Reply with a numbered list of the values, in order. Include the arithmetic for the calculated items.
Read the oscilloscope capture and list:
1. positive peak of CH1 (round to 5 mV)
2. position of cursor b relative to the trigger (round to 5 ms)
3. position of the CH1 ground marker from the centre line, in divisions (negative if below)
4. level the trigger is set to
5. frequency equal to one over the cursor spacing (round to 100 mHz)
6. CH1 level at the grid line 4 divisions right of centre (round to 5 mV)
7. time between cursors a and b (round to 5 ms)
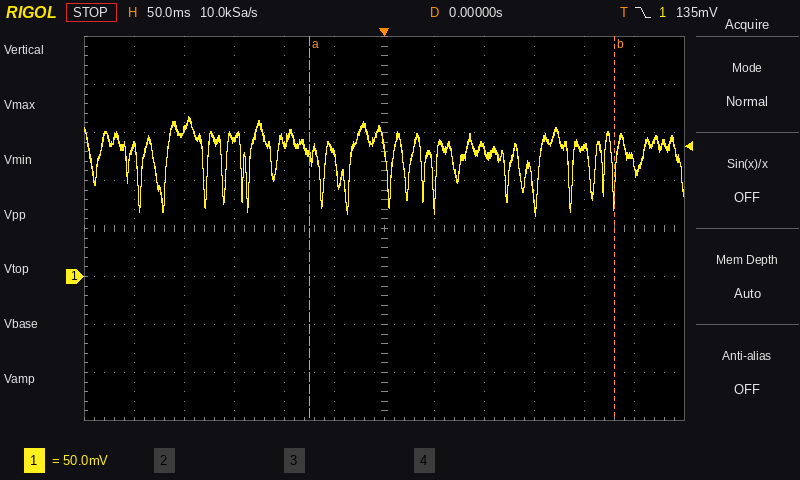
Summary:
1. 165 mV
2. +230 ms
3. -1.0 div
4. 135 mV
5. 1 / 305 ms ≈ 3.3 Hz
6. 135 mV
7. 305 ms
